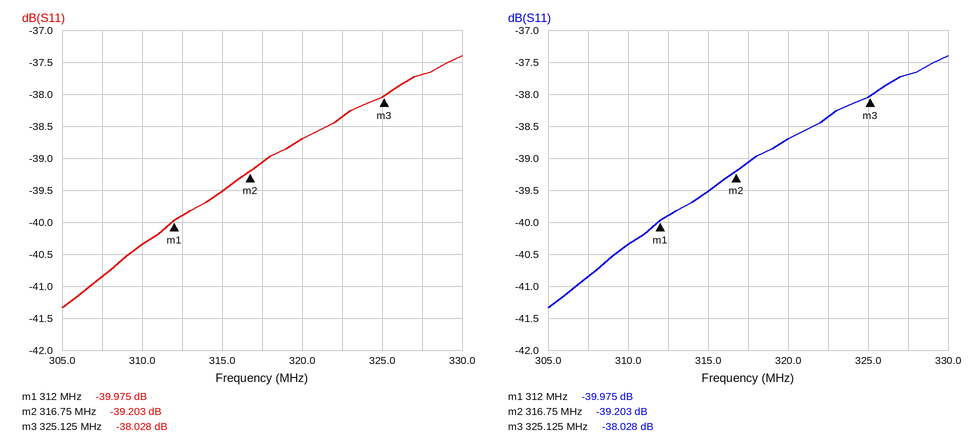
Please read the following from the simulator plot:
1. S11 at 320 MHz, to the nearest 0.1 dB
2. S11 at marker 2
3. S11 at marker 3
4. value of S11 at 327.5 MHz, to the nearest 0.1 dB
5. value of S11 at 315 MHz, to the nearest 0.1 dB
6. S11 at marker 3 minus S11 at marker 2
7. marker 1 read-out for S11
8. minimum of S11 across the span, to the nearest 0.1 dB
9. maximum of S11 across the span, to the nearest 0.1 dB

-38.7 dB
-39.203 dB
-38.028 dB
-37.7 dB
-39.5 dB
1.175 dB
-39.975 dB
-41.3 dB
-37.4 dB
